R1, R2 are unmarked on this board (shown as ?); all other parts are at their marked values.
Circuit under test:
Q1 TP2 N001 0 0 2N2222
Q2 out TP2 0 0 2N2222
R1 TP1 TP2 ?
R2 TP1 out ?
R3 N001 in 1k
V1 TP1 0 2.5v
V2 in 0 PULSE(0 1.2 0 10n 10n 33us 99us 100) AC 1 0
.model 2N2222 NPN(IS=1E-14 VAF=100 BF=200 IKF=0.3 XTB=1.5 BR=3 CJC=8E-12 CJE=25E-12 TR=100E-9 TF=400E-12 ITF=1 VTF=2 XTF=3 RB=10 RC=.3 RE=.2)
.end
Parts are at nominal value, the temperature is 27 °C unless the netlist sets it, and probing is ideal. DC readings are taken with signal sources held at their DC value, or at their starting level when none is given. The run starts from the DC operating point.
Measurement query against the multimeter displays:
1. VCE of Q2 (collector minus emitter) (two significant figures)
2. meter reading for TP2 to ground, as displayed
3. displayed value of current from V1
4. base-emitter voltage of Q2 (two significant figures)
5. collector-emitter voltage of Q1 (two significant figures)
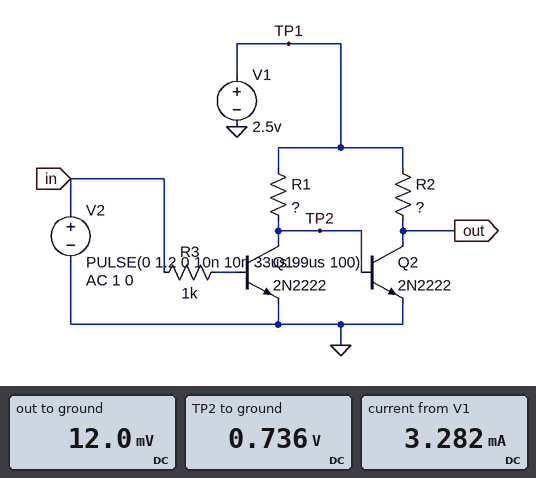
12 mV
0.736 V
3.282 mA
740 mV
740 mV
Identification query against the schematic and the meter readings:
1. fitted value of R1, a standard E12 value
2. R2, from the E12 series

820 Ω
2.2 kΩ
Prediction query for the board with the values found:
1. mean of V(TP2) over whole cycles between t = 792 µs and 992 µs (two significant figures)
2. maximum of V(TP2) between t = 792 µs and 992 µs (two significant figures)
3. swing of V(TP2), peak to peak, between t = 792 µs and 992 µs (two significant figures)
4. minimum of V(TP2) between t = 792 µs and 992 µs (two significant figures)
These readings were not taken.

500 mV
740 mV
710 mV
28 mV
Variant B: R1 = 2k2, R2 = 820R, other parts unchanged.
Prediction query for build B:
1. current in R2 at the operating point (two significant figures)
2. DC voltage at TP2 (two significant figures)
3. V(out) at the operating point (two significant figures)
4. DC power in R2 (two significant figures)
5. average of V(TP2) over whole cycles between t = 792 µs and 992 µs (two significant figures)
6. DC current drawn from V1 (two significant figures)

3.0 mA
710 mV
27 mV
7.5 mW
480 mV
3.8 mA
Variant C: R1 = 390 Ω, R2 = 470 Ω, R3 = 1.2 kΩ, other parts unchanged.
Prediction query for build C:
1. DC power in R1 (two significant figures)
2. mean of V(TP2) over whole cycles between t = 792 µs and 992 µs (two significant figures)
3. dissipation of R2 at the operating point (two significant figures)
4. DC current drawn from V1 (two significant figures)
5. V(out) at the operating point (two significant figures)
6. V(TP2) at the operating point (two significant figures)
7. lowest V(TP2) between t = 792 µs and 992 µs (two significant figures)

7.6 mW
540 mV
13 mW
9.7 mA
19 mV
780 mV
52 mV
